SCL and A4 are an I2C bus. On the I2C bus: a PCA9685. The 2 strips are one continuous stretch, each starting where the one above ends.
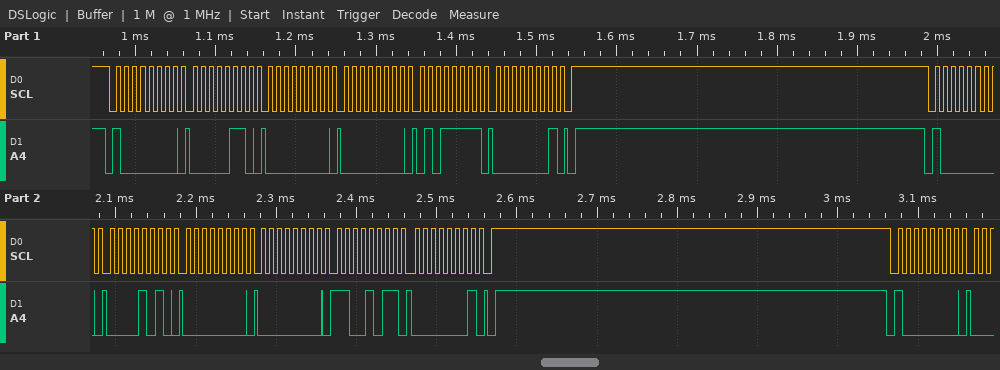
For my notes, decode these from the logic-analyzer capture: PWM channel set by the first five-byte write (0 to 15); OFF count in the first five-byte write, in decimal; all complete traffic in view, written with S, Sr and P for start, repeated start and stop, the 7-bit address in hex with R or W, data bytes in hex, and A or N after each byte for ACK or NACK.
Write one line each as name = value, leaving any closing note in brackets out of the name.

PWM channel set by the first five-byte write = 0
OFF count in the first five-byte write, in decimal = 351
all complete traffic in view, written with S, Sr and P for start, repeated start and stop, the 7-bit address in hex with R or W, data bytes in hex, and A or N after each byte for ACK or NACK = S 40W A 06 A 00 A 00 A 5F A 01 A P S 40W A 0A A 00 A 00 A CB A 01 A P S 40W A
